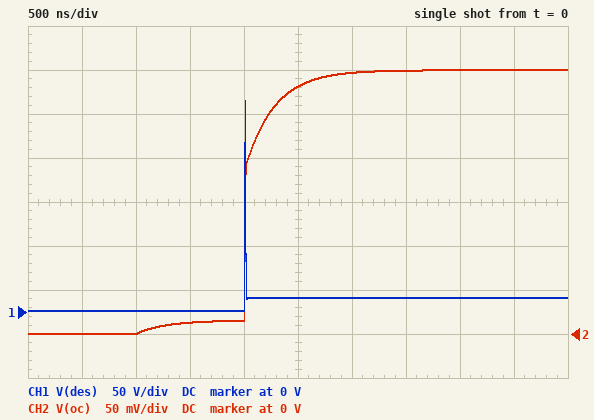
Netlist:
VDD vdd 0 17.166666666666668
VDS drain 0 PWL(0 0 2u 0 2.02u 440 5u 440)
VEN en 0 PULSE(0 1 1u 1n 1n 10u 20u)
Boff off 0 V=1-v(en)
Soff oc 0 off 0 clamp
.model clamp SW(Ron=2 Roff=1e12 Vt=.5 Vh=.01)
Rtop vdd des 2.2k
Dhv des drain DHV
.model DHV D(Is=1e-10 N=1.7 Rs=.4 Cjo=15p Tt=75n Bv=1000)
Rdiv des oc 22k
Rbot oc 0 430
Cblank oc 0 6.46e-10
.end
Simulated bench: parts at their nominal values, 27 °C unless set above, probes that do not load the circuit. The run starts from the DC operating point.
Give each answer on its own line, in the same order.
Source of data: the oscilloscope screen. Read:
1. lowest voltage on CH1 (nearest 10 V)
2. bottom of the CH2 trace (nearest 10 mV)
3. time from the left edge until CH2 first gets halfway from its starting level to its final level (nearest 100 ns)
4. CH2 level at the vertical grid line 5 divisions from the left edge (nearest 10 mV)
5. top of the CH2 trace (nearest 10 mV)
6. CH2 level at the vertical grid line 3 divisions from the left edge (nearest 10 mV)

0 V
0 V
2.0 µs
280 mV
300 mV
10 mV
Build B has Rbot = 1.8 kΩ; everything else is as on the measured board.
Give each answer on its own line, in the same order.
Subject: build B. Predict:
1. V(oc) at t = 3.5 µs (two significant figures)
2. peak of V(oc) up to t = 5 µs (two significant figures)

940 mV
1.1 V
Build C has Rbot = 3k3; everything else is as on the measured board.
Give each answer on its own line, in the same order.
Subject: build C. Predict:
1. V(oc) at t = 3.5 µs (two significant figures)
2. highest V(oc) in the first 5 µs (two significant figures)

1.2 V
1.7 V
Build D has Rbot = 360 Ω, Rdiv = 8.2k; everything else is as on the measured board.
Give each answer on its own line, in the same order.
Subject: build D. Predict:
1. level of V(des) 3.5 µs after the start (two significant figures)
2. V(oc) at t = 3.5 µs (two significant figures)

14 V
570 mV
